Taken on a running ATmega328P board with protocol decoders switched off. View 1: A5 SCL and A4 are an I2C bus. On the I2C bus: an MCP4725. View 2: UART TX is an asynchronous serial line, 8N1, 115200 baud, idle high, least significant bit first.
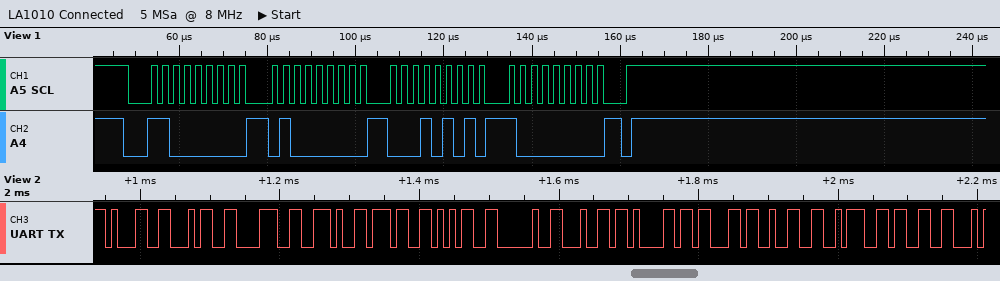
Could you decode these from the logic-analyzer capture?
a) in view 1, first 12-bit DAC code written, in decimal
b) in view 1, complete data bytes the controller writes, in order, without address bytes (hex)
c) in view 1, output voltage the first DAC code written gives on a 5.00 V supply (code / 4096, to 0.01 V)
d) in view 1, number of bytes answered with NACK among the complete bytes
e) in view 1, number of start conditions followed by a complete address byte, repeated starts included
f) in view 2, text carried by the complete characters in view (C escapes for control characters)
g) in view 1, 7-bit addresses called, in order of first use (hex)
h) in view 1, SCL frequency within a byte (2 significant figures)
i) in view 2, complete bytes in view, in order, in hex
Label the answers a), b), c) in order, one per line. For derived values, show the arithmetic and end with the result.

a) 344
b) 40 15 80
c) 344 / 4096 x 5.00 V = 0.42 V
d) 0
e) 1
f) "148.75 dac2:3"
g) 0x60
h) 400 kHz
i) 0x31 0x34 0x38 0x2E 0x37 0x35 0x20 0x64 0x61 0x63 0x32 0x3A 0x33
